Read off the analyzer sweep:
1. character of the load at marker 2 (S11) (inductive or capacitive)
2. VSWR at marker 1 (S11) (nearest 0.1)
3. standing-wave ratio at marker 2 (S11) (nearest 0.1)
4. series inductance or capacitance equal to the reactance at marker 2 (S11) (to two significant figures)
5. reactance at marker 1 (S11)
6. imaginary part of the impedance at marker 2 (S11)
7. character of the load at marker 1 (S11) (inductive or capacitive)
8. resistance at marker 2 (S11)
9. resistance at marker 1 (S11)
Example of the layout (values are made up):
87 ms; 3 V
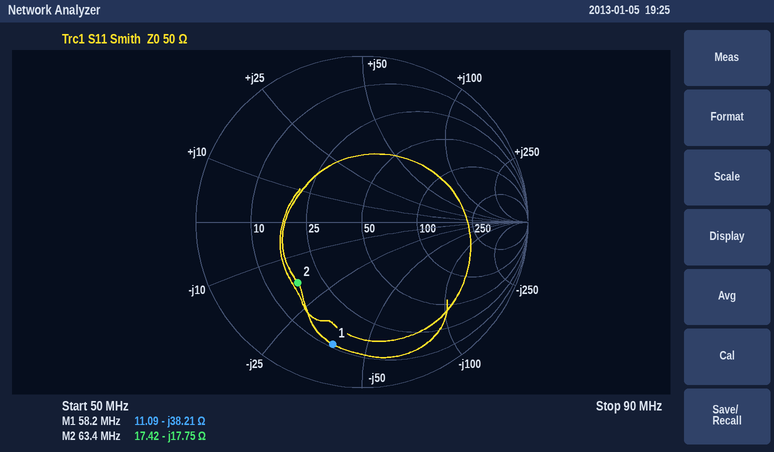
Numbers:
capacitive; 7.2; 3.3; 140 pF; -38.21 Ω; -17.75 Ω; capacitive; 17.42 Ω; 11.09 Ω
